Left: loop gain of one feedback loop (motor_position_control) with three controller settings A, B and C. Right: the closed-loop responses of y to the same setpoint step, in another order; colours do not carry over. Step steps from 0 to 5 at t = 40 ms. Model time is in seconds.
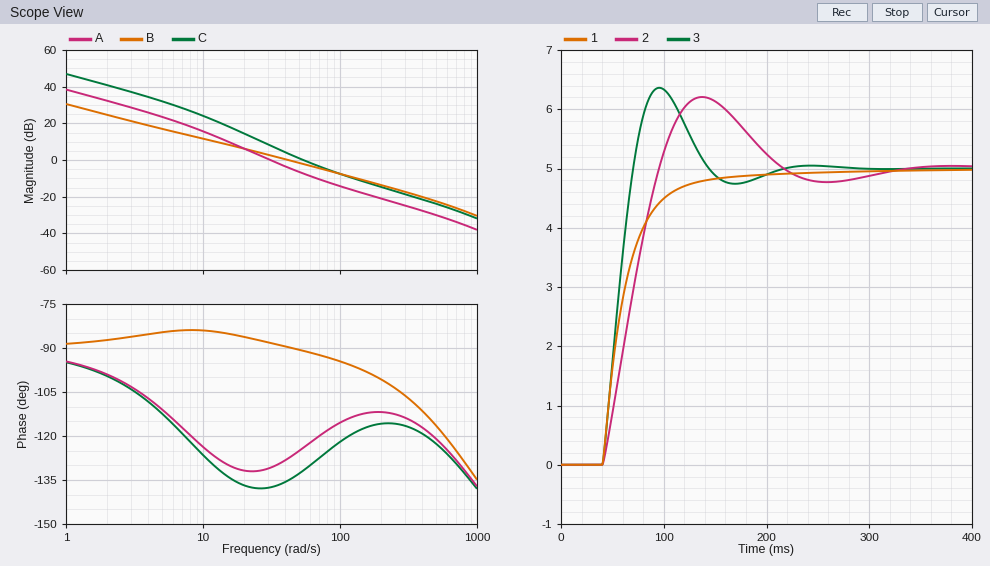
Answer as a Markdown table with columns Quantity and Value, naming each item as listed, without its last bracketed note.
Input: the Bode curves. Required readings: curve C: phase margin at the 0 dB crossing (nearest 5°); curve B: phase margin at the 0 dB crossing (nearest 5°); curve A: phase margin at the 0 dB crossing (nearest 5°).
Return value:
| Quantity | Value |
|---|---|
| curve C: phase margin at the 0 dB crossing | 50° |
| curve B: phase margin at the 0 dB crossing | 90° |
| curve A: phase margin at the 0 dB crossing | 50° |
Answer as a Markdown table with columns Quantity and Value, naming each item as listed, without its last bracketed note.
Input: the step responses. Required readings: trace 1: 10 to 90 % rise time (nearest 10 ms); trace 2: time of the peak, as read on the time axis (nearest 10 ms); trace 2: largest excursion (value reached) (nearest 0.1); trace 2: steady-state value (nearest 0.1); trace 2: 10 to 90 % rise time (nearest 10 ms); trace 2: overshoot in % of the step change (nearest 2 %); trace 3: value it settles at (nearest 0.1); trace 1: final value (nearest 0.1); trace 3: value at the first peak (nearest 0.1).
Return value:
| Quantity | Value |
|---|---|
| trace 1: 10 to 90 % rise time | 60 ms |
| trace 2: time of the peak, as read on the time axis | 140 ms |
| trace 2: largest excursion (value reached) | 6.2 |
| trace 2: steady-state value | 5.0 |
| trace 2: 10 to 90 % rise time | 40 ms |
| trace 2: overshoot in % of the step change | 24 % |
| trace 3: value it settles at | 5.0 |
| trace 1: final value | 5.0 |
| trace 3: value at the first peak | 6.4 |
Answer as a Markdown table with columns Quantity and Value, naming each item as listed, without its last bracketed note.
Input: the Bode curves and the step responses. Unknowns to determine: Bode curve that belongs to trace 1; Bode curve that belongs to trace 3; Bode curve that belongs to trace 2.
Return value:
| Quantity | Value |
|---|---|
| Bode curve that belongs to trace 1 | B |
| Bode curve that belongs to trace 3 | C |
| Bode curve that belongs to trace 2 | A |
